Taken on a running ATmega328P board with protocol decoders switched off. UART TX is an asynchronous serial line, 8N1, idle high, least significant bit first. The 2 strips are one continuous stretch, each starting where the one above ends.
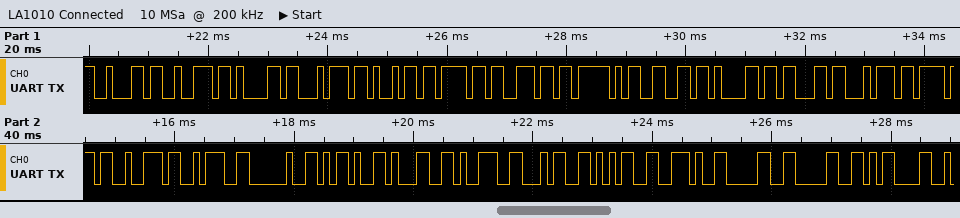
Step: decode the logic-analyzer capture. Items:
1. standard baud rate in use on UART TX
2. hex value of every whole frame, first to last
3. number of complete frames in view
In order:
9600 baud
62 72 61 74 69 6F 6E 5F 66 61 63 74 6F 72 3A 20 2D 31 39 34 35 2E 30 30 0D
25
